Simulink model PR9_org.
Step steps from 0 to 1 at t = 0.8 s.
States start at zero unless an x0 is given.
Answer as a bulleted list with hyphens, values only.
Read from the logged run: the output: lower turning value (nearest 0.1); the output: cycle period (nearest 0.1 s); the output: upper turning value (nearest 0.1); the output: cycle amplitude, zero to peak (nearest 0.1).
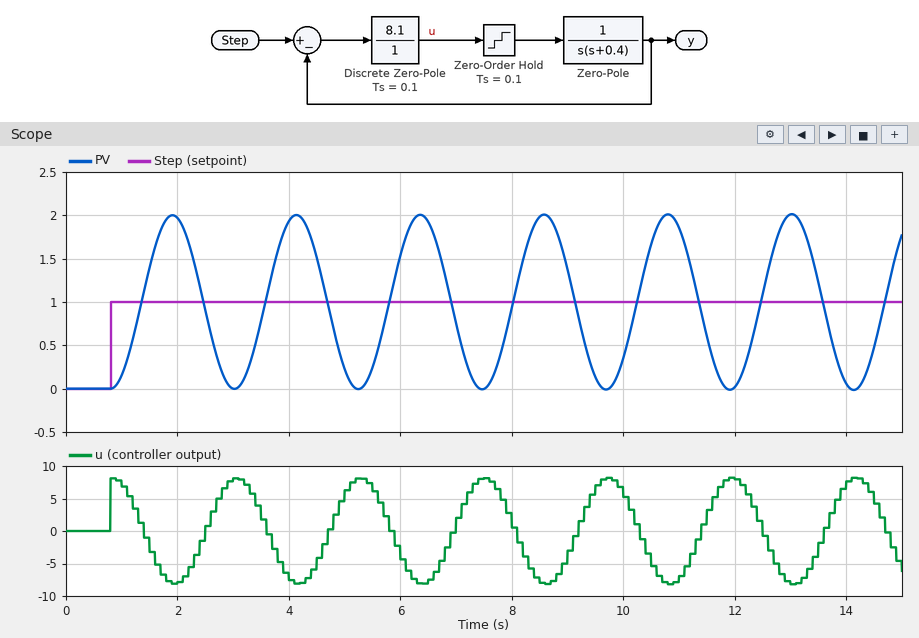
- 0.0
- 2.2 s
- 2.0
- 1.0
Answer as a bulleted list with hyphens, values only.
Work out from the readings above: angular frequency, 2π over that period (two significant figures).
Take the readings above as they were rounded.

- 2.9 rad/s
